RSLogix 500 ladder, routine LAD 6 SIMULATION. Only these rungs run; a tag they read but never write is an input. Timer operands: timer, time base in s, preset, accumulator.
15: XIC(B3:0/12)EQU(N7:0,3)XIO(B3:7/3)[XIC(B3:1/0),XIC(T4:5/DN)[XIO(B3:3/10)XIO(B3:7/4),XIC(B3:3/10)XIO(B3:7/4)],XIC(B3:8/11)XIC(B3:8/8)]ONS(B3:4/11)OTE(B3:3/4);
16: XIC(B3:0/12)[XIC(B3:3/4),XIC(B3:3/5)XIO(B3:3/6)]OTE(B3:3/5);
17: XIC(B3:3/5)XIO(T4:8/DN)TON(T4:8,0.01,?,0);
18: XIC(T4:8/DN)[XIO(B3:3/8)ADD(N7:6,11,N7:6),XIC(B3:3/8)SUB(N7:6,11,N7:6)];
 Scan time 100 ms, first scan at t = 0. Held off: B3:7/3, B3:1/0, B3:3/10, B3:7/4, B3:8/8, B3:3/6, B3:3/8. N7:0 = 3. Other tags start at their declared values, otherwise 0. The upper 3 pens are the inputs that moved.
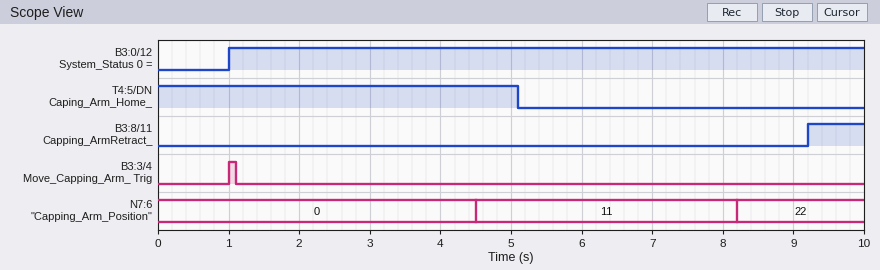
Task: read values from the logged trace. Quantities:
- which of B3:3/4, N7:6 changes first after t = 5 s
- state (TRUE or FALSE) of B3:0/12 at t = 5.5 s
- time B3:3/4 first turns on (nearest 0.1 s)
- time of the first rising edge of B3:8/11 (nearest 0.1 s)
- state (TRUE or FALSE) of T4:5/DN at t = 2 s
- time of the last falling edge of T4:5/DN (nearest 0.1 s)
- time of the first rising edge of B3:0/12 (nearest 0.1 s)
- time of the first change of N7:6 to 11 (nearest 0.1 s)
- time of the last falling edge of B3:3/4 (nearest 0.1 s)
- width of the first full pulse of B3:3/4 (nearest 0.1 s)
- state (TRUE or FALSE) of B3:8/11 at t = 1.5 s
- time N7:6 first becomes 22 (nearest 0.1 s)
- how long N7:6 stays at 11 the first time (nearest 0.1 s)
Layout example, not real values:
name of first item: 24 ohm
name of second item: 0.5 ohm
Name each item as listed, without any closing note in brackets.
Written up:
which of B3:3/4, N7:6 changes first after t = 5 s: N7:6
state (TRUE or FALSE) of B3:0/12 at t = 5.5 s: TRUE
time B3:3/4 first turns on: 1.0 s
time of the first rising edge of B3:8/11: 9.2 s
state (TRUE or FALSE) of T4:5/DN at t = 2 s: TRUE
time of the last falling edge of T4:5/DN: 5.1 s
time of the first rising edge of B3:0/12: 1.0 s
time of the first change of N7:6 to 11: 4.5 s
time of the last falling edge of B3:3/4: 1.1 s
width of the first full pulse of B3:3/4: 0.1 s
state (TRUE or FALSE) of B3:8/11 at t = 1.5 s: FALSE
time N7:6 first becomes 22: 8.2 s
how long N7:6 stays at 11 the first time: 3.7 s
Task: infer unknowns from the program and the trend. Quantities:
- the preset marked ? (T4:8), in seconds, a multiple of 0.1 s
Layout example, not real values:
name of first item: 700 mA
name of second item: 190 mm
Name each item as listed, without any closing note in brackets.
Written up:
the preset marked ? (T4:8), in seconds, a multiple of 0.1 s: 3.5 s
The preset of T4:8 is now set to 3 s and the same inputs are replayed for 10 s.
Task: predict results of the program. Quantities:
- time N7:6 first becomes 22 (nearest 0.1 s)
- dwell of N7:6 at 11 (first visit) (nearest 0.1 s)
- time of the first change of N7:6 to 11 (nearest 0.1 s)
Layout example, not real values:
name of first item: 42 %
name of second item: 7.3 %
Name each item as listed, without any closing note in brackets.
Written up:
time N7:6 first becomes 22: 7.2 s
dwell of N7:6 at 11 (first visit): 3.2 s
time of the first change of N7:6 to 11: 4.0 s
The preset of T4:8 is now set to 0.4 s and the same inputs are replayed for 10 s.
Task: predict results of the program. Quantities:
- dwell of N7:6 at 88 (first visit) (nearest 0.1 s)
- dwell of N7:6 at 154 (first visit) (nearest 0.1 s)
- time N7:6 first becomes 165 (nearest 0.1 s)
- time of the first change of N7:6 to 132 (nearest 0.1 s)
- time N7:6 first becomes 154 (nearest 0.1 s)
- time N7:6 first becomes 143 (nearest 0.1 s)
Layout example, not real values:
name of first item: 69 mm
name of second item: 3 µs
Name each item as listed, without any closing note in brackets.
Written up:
dwell of N7:6 at 88 (first visit): 0.6 s
dwell of N7:6 at 154 (first visit): 0.6 s
time N7:6 first becomes 165: 9.8 s
time of the first change of N7:6 to 132: 8.0 s
time N7:6 first becomes 154: 9.2 s
time N7:6 first becomes 143: 8.6 s
